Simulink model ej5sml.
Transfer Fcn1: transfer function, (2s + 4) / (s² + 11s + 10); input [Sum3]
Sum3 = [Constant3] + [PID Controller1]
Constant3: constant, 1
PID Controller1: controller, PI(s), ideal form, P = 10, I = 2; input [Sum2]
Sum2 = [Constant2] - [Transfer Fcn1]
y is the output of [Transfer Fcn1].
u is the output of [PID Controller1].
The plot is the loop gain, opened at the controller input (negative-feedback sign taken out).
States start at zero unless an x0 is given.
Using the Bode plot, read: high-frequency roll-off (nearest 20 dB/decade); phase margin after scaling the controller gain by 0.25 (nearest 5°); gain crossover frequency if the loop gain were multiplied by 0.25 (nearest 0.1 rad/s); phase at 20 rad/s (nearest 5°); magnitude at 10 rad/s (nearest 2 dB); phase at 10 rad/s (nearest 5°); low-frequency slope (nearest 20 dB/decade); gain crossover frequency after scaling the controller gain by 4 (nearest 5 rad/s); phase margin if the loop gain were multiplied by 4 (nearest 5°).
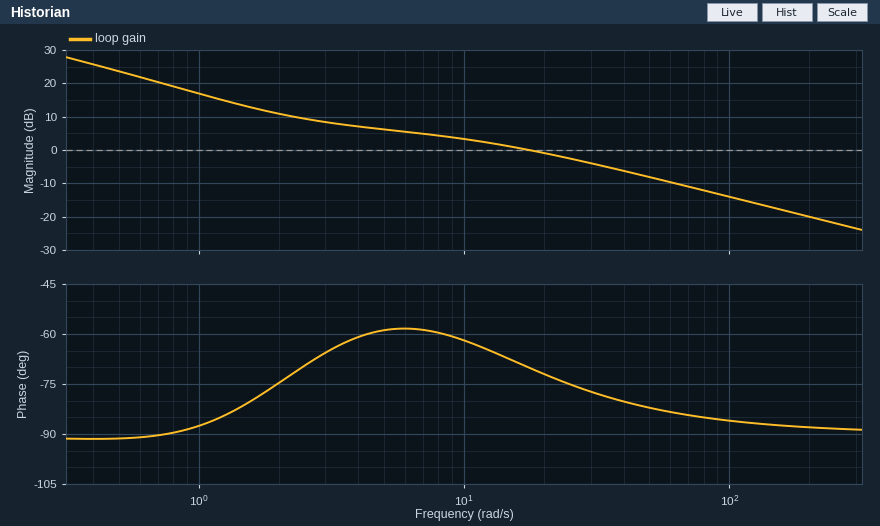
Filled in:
-20 dB/decade
100°
1.7 rad/s
-70°
4 dB
-60°
-20 dB/decade
80 rad/s
95°
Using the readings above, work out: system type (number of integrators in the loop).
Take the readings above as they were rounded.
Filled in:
1
